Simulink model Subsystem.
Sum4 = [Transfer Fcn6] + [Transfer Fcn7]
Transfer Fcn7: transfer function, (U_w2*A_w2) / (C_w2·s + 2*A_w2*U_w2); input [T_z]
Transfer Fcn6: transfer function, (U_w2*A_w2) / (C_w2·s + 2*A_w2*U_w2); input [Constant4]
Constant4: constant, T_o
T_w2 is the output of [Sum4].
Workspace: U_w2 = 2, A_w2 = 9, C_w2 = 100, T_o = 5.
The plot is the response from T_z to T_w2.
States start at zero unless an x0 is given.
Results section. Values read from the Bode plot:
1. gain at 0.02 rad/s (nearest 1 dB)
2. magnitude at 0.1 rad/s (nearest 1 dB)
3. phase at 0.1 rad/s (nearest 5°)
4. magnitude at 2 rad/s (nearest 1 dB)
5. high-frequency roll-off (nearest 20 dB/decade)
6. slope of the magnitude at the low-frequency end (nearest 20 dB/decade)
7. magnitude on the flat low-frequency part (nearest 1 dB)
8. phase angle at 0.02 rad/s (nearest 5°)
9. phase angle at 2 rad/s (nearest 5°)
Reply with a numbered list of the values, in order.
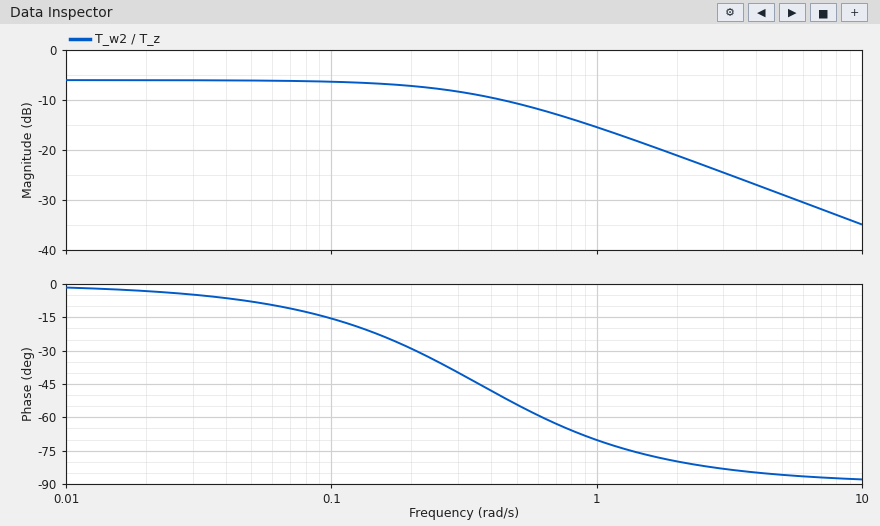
1. -6 dB
2. -6 dB
3. -15°
4. -21 dB
5. -20 dB/decade
6. 0 dB/decade
7. -6 dB
8. -5°
9. -80°
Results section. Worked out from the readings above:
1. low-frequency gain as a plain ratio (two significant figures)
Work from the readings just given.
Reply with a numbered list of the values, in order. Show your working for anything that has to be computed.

1. 10^(-6 / 20) = 0.50
